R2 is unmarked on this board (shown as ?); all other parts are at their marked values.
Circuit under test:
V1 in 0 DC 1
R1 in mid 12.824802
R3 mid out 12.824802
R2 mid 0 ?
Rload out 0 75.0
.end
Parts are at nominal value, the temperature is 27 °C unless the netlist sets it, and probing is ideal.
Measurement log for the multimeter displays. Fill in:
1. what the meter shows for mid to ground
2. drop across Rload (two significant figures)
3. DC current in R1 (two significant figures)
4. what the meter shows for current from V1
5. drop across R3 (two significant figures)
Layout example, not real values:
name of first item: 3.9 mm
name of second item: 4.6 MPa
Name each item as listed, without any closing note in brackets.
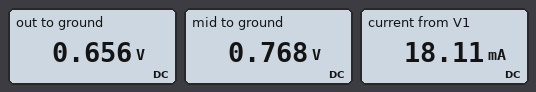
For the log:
what the meter shows for mid to ground: 0.768 V
drop across Rload: 660 mV
DC current in R1: 18 mA
what the meter shows for current from V1: 18.11 mA
drop across R3: 110 mV
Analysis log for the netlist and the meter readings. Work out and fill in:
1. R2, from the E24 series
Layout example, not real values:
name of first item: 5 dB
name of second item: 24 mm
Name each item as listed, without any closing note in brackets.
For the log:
R2, from the E24 series: 82 Ω
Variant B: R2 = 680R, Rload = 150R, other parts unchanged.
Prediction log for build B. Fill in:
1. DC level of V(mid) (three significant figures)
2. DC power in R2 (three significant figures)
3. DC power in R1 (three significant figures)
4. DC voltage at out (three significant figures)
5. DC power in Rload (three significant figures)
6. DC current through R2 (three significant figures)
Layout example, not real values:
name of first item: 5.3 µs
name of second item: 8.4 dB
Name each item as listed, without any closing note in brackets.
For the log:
DC level of V(mid): 911 mV
DC power in R2: 1.22 mW
DC power in R1: 617 µW
DC voltage at out: 839 mV
DC power in Rload: 4.70 mW
DC current through R2: 1.34 mA
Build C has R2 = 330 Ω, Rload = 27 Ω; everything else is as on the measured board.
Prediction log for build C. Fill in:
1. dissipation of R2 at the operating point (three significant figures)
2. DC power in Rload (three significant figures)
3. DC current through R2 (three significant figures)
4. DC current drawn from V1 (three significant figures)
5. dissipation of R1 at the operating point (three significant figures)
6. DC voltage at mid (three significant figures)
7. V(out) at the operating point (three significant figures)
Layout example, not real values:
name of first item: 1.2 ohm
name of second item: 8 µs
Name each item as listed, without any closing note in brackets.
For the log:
dissipation of R2 at the operating point: 1.64 mW
DC power in Rload: 9.19 mW
DC current through R2: 2.23 mA
DC current drawn from V1: 20.7 mA
dissipation of R1 at the operating point: 5.48 mW
DC voltage at mid: 735 mV
V(out) at the operating point: 498 mV
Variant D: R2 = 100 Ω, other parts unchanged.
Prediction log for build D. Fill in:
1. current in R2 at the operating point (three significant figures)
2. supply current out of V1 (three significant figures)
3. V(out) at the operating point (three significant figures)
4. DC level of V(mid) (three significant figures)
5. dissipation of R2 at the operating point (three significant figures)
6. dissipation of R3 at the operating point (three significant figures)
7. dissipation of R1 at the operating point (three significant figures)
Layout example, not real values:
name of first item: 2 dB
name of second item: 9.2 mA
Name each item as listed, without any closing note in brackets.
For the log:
current in R2 at the operating point: 7.85 mA
supply current out of V1: 16.8 mA
V(out) at the operating point: 670 mV
DC level of V(mid): 785 mV
dissipation of R2 at the operating point: 6.16 mW
dissipation of R3 at the operating point: 1.02 mW
dissipation of R1 at the operating point: 3.61 mW
